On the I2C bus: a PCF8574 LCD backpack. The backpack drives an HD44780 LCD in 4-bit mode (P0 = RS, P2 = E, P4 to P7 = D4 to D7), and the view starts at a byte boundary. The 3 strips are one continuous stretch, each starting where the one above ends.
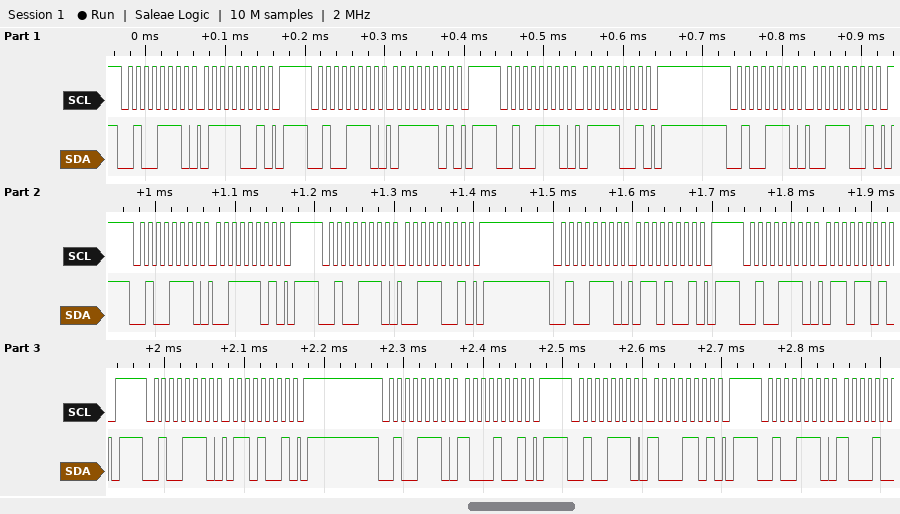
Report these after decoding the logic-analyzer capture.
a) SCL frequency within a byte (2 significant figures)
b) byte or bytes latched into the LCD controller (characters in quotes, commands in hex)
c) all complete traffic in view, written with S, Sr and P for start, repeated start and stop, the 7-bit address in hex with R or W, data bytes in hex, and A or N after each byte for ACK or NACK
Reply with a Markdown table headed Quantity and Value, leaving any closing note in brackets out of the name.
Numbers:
| Quantity | Value |
|---|---|
| SCL frequency within a byte | 100 kHz |
| byte or bytes latched into the LCD controller | 's' |
| all complete traffic in view, written with S, Sr and P for start, repeated start and stop, the 7-bit address in hex with R or W, data bytes in hex, and A or N after each byte for ACK or NACK | S 27W A 79 A P S 27W A 7D A P S 27W A 79 A P S 27W A 39 A P S 27W A 3D A P S 27W A 39 A P S 27W A 69 A P S 27W A 6D A P S 27W A 69 A P S 27W A 89 A P S 27W A 8D A P S 27W A |
